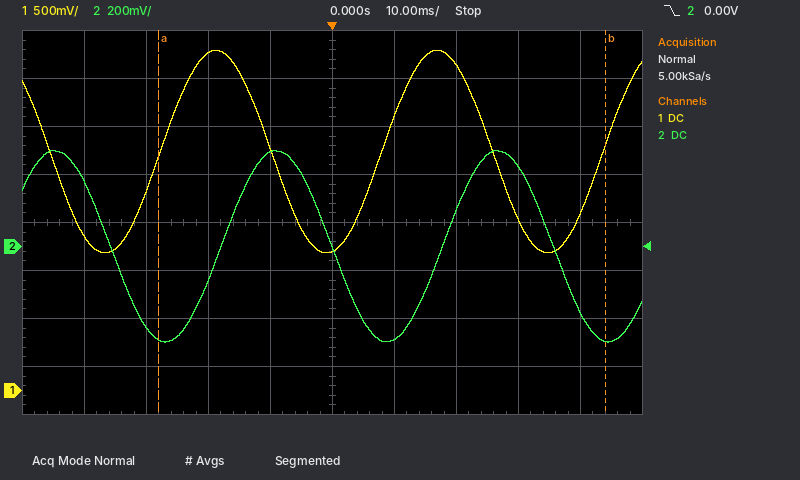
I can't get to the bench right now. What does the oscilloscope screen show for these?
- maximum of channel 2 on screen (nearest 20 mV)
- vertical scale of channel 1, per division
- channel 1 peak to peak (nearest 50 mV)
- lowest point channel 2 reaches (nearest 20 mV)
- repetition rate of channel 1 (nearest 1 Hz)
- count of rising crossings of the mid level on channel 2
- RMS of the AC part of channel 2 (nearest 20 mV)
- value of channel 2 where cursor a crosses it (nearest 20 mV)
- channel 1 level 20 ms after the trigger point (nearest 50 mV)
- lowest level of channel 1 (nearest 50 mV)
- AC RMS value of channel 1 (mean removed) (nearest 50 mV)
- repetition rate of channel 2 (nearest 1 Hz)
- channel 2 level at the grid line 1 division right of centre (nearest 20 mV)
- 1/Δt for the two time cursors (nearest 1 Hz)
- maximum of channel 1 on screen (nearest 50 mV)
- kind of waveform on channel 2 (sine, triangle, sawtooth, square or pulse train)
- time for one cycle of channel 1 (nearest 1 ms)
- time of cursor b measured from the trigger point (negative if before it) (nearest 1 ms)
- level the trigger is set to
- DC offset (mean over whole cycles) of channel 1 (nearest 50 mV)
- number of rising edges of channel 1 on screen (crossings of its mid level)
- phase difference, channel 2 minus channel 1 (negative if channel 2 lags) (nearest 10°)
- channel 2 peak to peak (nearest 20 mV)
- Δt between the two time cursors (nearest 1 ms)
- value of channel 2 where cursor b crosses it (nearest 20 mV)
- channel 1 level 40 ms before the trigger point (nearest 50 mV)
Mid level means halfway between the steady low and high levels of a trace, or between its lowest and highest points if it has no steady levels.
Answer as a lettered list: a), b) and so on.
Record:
a) 400 mV
b) 500 mV
c) 2.10 V
d) -400 mV
e) 28 Hz
f) 2
g) 280 mV
h) -380 mV
i) 3.40 V
j) 1.45 V
k) 750 mV
l) 28 Hz
m) -380 mV
n) 14 Hz
o) 3.55 V
p) sine
q) 36 ms
r) +44 ms
s) 0.00 V
t) 2.50 V
u) 3
v) -100°
w) 800 mV
x) 72 ms
y) -400 mV
z) 1.60 V
